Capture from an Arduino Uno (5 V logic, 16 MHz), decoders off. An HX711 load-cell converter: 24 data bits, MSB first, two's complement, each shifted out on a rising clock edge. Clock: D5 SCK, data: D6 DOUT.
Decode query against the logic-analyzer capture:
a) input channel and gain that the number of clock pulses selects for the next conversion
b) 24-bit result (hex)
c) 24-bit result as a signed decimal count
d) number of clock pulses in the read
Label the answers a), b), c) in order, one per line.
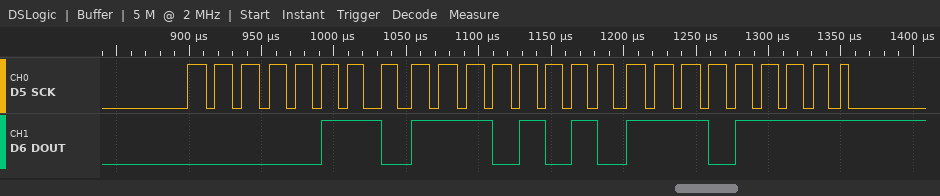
a) channel A, gain 128
b) 0x06EAEF
c) 453359
d) 25
